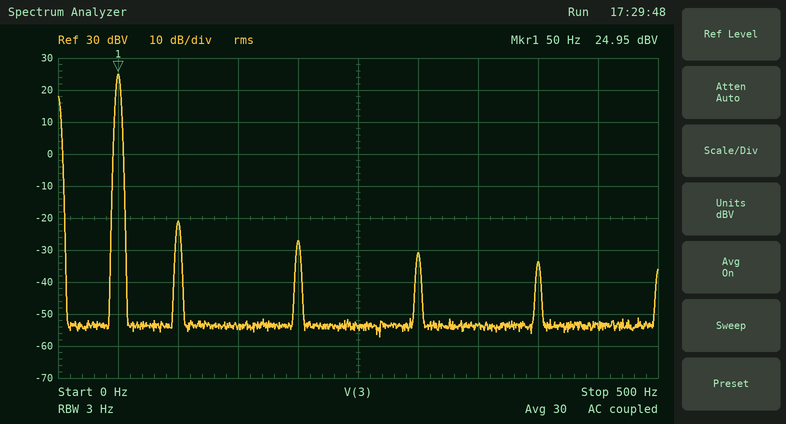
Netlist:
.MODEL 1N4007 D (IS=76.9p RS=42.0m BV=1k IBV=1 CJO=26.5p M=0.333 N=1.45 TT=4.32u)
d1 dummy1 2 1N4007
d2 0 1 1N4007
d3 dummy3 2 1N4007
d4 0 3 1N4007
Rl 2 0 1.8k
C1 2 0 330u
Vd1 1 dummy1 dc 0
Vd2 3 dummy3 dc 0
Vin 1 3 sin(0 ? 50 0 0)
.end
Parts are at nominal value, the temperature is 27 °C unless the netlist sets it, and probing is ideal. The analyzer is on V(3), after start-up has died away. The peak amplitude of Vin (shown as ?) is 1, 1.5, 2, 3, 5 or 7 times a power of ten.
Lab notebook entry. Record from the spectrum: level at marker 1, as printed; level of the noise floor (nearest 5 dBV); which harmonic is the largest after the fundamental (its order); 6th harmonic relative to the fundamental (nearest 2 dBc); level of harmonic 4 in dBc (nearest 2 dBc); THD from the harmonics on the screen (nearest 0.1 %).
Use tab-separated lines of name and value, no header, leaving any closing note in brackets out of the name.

level at marker 1, as printed	24.95 dBV
level of the noise floor	-55 dBV
which harmonic is the largest after the fundamental	2
6th harmonic relative to the fundamental	-56 dBc
level of harmonic 4 in dBc	-52 dBc
THD from the harmonics on the screen	0.6 %
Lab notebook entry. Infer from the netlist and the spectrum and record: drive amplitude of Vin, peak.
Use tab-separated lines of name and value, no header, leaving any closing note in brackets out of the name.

drive amplitude of Vin, peak	50 V
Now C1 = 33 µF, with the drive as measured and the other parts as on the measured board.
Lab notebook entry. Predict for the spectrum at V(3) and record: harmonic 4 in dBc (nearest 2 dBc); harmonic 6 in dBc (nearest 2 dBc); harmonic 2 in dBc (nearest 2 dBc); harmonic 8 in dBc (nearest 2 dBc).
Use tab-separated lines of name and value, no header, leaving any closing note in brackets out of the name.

harmonic 4 in dBc	-34 dBc
harmonic 6 in dBc	-38 dBc
harmonic 2 in dBc	-26 dBc
harmonic 8 in dBc	-44 dBc
